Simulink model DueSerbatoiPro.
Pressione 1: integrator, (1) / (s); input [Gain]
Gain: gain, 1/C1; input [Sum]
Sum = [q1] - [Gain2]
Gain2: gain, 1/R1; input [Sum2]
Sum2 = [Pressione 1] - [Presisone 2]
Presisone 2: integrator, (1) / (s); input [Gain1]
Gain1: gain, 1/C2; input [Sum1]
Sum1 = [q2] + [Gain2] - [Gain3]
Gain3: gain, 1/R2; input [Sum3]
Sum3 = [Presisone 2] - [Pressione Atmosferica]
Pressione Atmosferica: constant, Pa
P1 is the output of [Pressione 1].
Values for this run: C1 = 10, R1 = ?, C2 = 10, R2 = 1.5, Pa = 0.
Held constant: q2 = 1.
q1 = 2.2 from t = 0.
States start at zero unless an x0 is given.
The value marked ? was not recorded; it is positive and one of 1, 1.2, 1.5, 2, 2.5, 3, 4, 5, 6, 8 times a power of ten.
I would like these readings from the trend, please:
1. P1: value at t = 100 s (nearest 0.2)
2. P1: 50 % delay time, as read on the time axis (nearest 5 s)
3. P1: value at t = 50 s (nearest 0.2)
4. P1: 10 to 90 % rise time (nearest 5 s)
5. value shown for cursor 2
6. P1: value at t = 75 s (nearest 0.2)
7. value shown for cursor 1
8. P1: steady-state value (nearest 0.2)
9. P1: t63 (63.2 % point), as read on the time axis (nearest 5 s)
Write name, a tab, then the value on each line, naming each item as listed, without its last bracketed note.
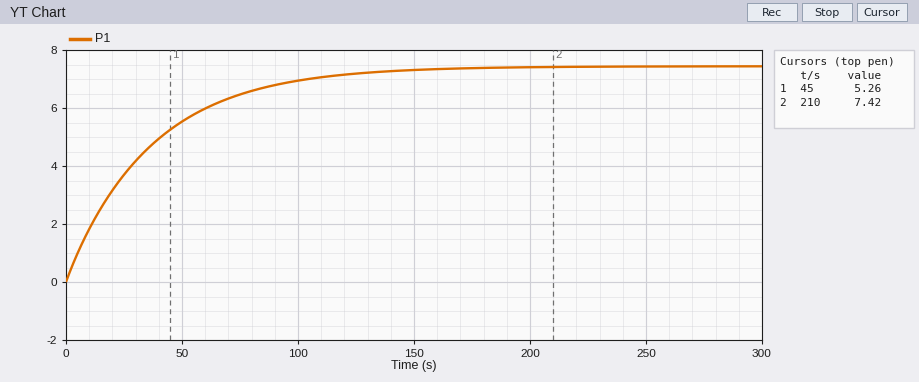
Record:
P1: value at t = 100 s	7.0
P1: 50 % delay time, as read on the time axis	25 s
P1: value at t = 50 s	5.6
P1: 10 to 90 % rise time	80 s
value shown for cursor 2	7.42
P1: value at t = 75 s	6.4
value shown for cursor 1	5.26
P1: steady-state value	7.4
P1: t63 (63.2 % point), as read on the time axis	35 s
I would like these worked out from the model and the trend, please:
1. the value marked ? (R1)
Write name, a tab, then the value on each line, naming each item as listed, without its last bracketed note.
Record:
the value marked ?	1.2
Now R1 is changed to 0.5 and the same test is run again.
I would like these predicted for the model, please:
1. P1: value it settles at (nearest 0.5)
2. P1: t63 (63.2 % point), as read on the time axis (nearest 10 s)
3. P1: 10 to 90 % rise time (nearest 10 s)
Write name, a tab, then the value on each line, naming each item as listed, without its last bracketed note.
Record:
P1: value it settles at	6.0
P1: t63 (63.2 % point), as read on the time axis	30 s
P1: 10 to 90 % rise time	70 s
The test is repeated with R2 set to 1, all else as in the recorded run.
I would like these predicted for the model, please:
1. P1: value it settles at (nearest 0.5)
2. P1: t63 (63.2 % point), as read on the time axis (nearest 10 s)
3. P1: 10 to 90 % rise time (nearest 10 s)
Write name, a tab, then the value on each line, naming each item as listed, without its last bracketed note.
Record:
P1: value it settles at	6.0
P1: t63 (63.2 % point), as read on the time axis	30 s
P1: 10 to 90 % rise time	60 s
